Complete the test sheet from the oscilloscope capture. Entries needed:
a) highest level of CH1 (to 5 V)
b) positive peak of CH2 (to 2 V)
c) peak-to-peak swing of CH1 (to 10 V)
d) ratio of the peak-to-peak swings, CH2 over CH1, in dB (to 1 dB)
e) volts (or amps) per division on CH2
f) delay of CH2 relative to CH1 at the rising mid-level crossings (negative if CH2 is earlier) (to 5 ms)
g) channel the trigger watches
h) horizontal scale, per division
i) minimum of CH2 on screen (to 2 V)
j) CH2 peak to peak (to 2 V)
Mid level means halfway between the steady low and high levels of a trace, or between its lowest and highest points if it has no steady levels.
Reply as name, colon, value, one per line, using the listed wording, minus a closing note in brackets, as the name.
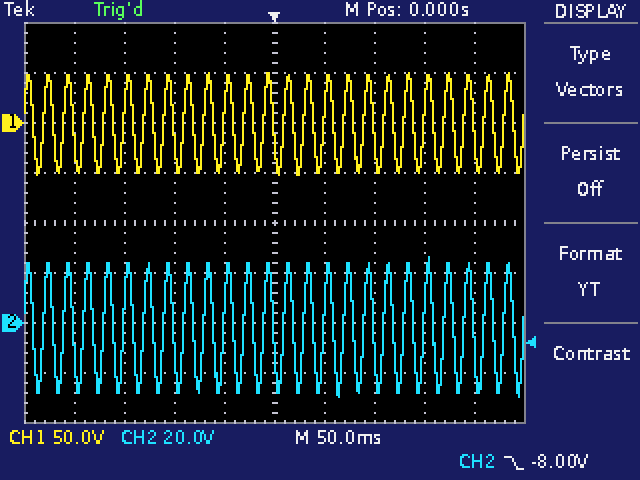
highest level of CH1: 50 V
positive peak of CH2: 26 V
peak-to-peak swing of CH1: 100 V
ratio of the peak-to-peak swings, CH2 over CH1, in dB: -5 dB
volts (or amps) per division on CH2: 20 V
delay of CH2 relative to CH1 at the rising mid-level crossings (negative if CH2 is earlier): 0 ms
channel the trigger watches: CH2
horizontal scale, per division: 50 ms
minimum of CH2 on screen: -30 V
CH2 peak to peak: 56 V
